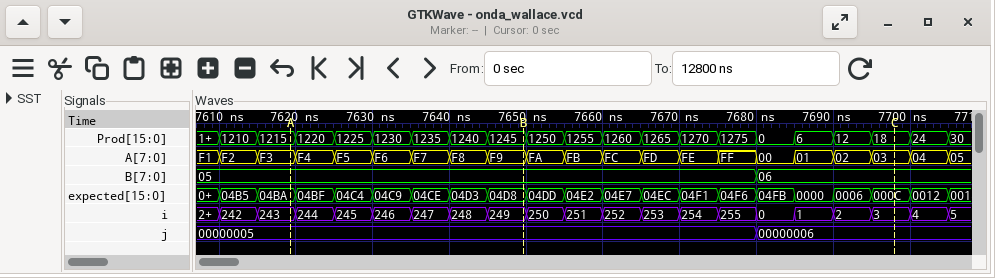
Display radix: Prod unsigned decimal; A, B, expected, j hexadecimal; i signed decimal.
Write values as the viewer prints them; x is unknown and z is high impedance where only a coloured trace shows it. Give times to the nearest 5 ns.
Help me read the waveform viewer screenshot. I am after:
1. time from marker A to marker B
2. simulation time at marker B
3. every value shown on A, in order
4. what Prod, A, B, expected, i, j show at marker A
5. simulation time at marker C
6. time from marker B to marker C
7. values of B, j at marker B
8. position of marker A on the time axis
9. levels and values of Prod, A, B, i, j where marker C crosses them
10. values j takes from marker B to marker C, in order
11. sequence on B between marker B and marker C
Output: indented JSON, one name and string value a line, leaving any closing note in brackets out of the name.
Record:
{
  "time from marker A to marker B": "30 ns",
  "simulation time at marker B": "7650 ns",
  "every value shown on A, in order": "F1, F2, F3, F4, F5, F6, F7, F8, F9, FA, FB, FC, FD, FE, FF, 00, 01, 02, 03, 04, 05",
  "what Prod, A, B, expected, i, j show at marker A": "Prod=1215, A=F3, B=05, expected=04BA, i=243, j=00000005",
  "simulation time at marker C": "7700 ns",
  "time from marker B to marker C": "50 ns",
  "values of B, j at marker B": "B=05, j=00000005",
  "position of marker A on the time axis": "7620 ns",
  "levels and values of Prod, A, B, i, j where marker C crosses them": "Prod=18, A=03, B=06, i=3, j=00000006",
  "values j takes from marker B to marker C, in order": "00000005, 00000006",
  "sequence on B between marker B and marker C": "05, 06"
}
